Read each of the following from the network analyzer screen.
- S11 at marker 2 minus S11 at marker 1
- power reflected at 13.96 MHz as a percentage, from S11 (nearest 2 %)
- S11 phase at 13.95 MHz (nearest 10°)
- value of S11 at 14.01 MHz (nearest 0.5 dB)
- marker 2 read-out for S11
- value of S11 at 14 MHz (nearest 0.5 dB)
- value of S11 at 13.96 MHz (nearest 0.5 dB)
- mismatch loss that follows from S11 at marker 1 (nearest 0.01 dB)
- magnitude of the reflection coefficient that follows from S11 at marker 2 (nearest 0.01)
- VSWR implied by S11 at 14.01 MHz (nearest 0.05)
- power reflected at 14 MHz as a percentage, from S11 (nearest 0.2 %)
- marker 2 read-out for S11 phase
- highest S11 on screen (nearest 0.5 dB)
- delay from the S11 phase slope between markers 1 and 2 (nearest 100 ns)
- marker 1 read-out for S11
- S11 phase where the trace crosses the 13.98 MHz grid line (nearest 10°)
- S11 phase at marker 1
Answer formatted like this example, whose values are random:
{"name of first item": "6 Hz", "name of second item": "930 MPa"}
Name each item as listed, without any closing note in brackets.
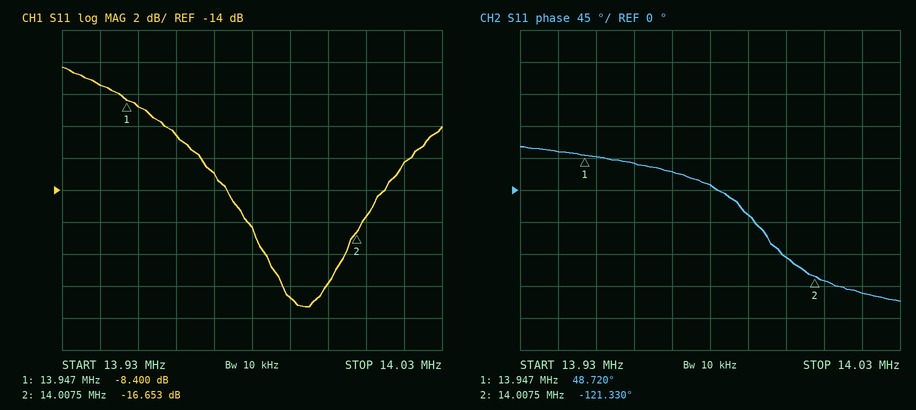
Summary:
{"S11 at marker 2 minus S11 at marker 1": "-8.253 dB", "power reflected at 13.96 MHz as a percentage, from S11": "8 %", "S11 phase at 13.95 MHz": "50°", "value of S11 at 14.01 MHz": "-15.5 dB", "marker 2 read-out for S11": "-16.653 dB", "value of S11 at 14 MHz": "-20.0 dB", "value of S11 at 13.96 MHz": "-10.5 dB", "mismatch loss that follows from S11 at marker 1": "0.68 dB", "magnitude of the reflection coefficient that follows from S11 at marker 2": "0.15", "VSWR implied by S11 at 14.01 MHz": "1.40", "power reflected at 14 MHz as a percentage, from S11": "1.0 %", "marker 2 read-out for S11 phase": "-121.330°", "highest S11 on screen": "-6.5 dB", "delay from the S11 phase slope between markers 1 and 2": "7.8 µs", "marker 1 read-out for S11": "-8.400 dB", "S11 phase where the trace crosses the 13.98 MHz grid line": "10°", "S11 phase at marker 1": "48.720°"}
